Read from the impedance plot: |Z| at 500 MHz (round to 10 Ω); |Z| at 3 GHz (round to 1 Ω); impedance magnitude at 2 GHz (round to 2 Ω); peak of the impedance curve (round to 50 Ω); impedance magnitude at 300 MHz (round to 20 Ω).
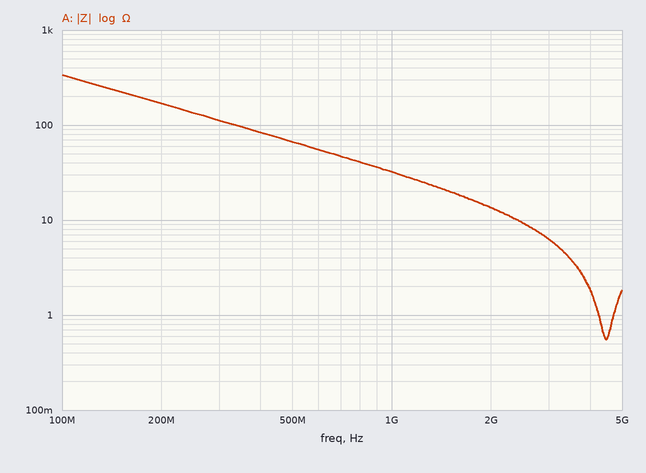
70 Ω
6 Ω
14 Ω
350 Ω
120 Ω
